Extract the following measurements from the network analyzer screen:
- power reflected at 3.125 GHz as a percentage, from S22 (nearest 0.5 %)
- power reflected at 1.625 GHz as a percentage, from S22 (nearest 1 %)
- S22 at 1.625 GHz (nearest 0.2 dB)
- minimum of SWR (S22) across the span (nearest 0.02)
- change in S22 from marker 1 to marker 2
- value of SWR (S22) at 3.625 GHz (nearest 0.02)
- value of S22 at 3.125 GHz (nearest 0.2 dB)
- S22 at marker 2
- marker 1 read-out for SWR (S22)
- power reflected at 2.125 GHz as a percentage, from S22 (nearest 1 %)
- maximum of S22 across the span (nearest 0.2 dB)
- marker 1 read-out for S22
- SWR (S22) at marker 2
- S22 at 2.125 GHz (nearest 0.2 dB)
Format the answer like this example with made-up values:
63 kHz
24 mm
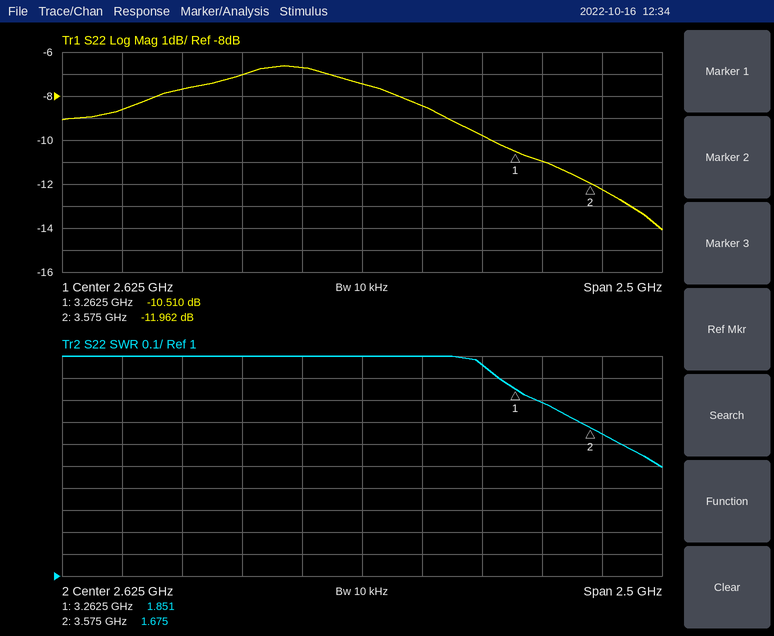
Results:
10.5 %
14 %
-8.6 dB
1.50
-1.452 dB
1.64
-9.8 dB
-11.962 dB
1.851
20 %
-6.6 dB
-10.510 dB
1.675
-7.0 dB
